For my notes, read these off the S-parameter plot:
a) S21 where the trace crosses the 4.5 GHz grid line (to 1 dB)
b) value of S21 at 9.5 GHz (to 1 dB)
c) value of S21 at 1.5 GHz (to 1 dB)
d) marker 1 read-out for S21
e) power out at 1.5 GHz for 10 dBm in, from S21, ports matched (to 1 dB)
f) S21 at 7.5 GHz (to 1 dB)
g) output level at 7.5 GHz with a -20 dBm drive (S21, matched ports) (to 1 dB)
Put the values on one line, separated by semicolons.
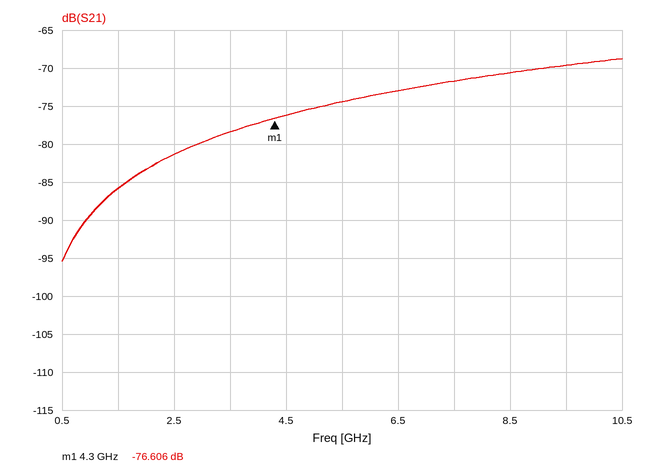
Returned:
-76 dB; -70 dB; -86 dB; -76.606 dB; -76 dBm; -72 dB; -92 dBm
